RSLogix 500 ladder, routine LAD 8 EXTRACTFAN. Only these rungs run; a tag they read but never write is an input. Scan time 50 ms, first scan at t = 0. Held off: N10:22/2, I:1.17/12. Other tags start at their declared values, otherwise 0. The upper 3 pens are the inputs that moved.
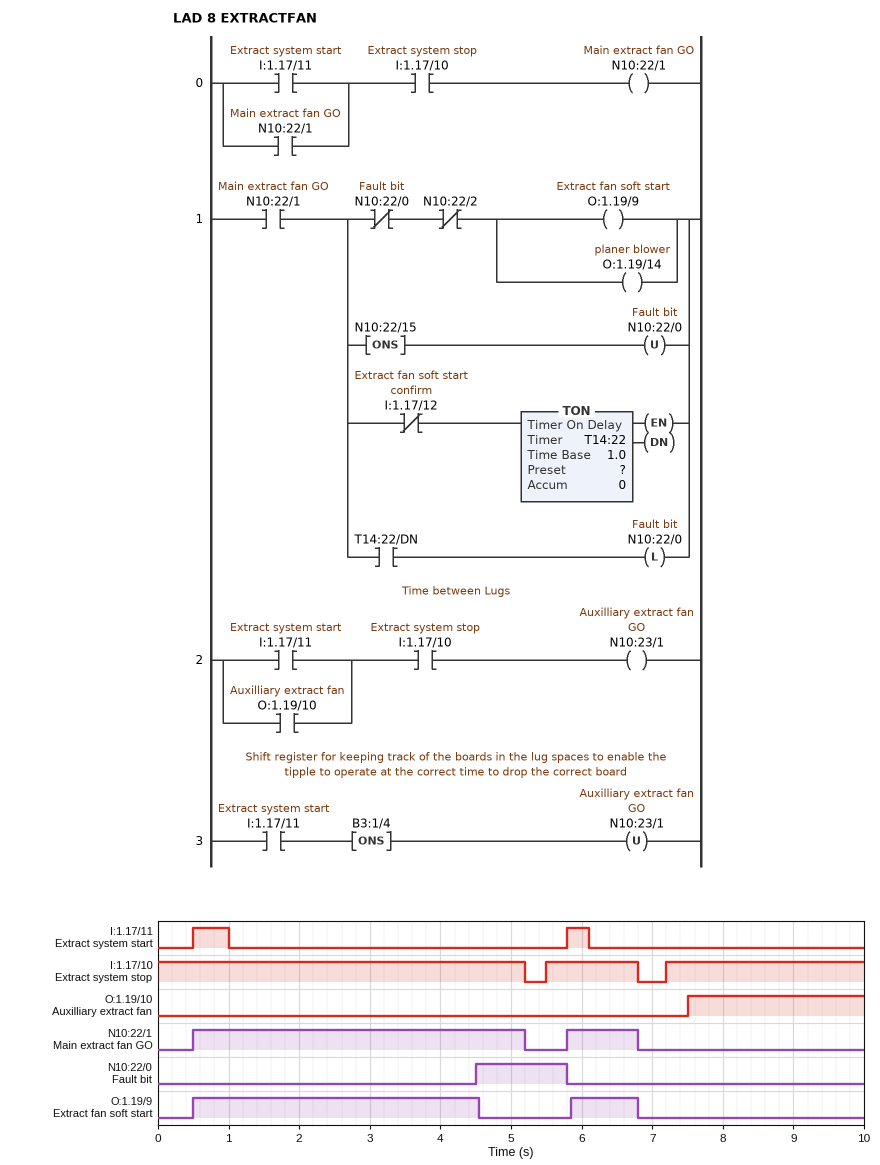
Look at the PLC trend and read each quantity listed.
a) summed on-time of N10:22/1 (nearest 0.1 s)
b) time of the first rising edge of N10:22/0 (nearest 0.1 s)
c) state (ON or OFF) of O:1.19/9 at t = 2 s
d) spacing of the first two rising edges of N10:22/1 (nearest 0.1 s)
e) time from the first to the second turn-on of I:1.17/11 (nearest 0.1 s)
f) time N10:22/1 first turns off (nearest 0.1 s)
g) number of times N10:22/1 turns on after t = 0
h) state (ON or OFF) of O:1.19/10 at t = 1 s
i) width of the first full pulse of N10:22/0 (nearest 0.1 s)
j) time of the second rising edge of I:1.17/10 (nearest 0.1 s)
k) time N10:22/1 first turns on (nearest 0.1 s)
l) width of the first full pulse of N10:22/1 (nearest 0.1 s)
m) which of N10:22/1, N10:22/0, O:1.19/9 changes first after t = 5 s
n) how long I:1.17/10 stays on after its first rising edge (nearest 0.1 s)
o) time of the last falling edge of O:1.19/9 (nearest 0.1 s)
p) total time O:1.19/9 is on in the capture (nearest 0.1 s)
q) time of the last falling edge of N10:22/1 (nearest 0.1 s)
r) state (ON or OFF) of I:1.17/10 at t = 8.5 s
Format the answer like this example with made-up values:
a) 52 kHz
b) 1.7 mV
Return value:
a) 5.7 s
b) 4.5 s
c) ON
d) 5.3 s
e) 5.3 s
f) 5.2 s
g) 2
h) OFF
i) 1.3 s
j) 7.2 s
k) 0.5 s
l) 4.7 s
m) N10:22/1
n) 1.3 s
o) 6.8 s
p) 5.0 s
q) 6.8 s
r) ON
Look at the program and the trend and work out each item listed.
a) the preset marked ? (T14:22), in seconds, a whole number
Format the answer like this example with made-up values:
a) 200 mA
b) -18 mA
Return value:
a) 4 s
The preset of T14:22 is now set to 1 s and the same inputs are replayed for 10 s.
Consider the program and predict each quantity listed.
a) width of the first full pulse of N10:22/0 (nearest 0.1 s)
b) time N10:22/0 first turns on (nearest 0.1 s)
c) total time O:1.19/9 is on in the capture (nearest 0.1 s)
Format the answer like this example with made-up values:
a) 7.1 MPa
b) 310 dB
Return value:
a) 4.3 s
b) 1.5 s
c) 2.0 s
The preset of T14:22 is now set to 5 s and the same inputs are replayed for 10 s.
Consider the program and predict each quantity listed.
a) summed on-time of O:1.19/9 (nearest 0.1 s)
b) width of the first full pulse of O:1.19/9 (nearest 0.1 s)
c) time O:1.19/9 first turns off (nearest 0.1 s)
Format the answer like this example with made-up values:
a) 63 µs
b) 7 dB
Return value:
a) 5.7 s
b) 4.7 s
c) 5.2 s
